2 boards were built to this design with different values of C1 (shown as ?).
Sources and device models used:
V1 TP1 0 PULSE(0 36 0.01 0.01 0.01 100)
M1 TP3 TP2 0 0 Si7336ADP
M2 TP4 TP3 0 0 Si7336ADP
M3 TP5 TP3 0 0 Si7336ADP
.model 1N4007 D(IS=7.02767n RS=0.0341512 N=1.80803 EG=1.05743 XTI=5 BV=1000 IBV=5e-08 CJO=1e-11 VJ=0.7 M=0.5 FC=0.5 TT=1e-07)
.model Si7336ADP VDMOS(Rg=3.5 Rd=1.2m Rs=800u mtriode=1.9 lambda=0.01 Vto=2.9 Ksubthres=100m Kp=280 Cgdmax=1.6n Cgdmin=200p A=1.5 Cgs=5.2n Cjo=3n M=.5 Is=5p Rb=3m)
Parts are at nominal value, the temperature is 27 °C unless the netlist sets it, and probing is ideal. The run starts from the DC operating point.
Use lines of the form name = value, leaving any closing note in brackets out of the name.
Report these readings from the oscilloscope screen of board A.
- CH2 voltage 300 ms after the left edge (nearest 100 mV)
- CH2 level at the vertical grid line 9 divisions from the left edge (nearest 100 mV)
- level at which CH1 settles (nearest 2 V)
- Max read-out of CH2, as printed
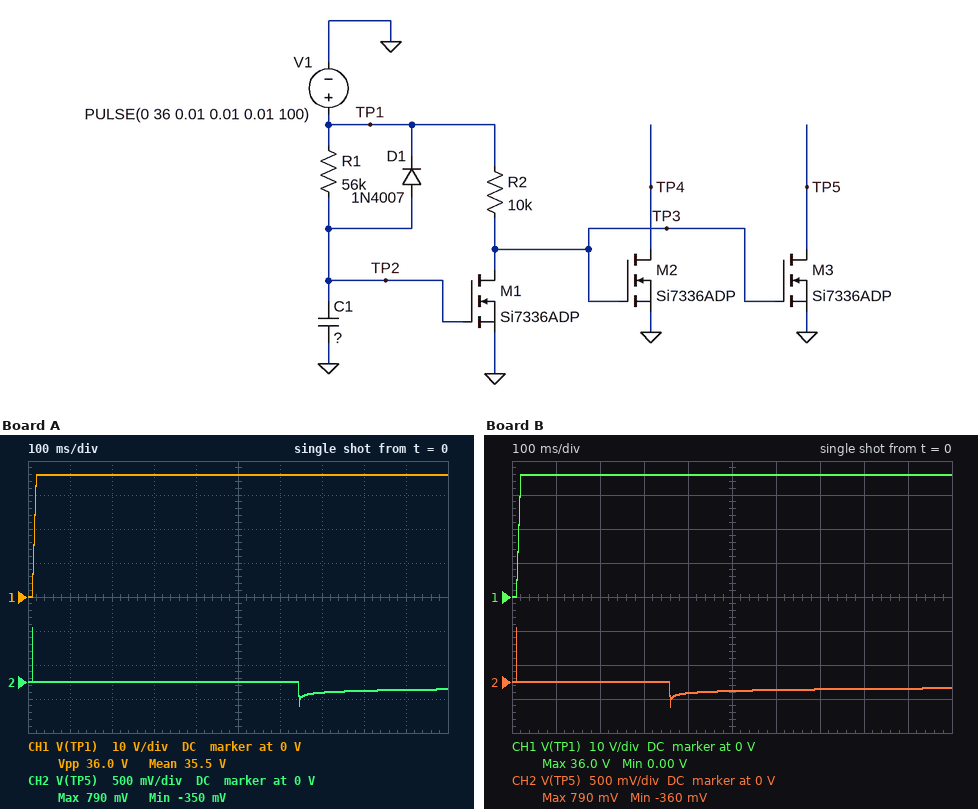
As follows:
CH2 voltage 300 ms after the left edge = 0 V
CH2 level at the vertical grid line 9 divisions from the left edge = -100 mV
level at which CH1 settles = 36 V
Max read-out of CH2, as printed = 790 mV
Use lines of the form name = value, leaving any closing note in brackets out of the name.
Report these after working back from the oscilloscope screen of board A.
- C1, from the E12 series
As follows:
C1, from the E12 series = 150 µF
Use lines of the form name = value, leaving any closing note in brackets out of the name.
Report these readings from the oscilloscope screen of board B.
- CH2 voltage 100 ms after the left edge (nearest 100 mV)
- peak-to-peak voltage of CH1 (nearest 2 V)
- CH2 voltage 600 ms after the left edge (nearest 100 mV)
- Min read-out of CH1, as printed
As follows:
CH2 voltage 100 ms after the left edge = 0 V
peak-to-peak voltage of CH1 = 36 V
CH2 voltage 600 ms after the left edge = -100 mV
Min read-out of CH1, as printed = 0.00 V
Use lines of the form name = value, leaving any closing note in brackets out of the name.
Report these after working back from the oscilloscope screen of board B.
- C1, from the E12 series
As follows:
C1, from the E12 series = 82 µF
